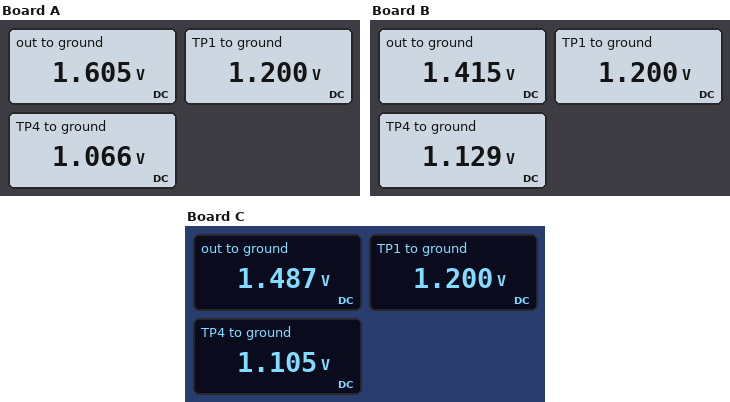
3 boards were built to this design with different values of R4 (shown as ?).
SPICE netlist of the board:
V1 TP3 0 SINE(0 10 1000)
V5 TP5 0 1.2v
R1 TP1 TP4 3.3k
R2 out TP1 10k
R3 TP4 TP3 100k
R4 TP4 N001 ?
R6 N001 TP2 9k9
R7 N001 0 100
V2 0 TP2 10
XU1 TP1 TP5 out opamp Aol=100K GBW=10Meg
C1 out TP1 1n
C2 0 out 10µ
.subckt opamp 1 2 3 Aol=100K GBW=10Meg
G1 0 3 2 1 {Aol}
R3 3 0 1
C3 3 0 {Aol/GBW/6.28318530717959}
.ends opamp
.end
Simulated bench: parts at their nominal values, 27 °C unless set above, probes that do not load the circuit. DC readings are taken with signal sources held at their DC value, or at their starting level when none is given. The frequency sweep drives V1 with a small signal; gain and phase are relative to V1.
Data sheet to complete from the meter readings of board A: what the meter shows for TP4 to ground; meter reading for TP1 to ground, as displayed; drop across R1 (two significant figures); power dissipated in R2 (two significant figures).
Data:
1.066 V
1.200 V
130 mV
16 µW
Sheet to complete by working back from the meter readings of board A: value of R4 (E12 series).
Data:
39 kΩ
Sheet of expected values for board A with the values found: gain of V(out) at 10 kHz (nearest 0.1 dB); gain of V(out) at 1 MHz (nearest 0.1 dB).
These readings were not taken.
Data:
-22.4 dB
-57.0 dB
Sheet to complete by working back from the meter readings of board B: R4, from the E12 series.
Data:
120 kΩ
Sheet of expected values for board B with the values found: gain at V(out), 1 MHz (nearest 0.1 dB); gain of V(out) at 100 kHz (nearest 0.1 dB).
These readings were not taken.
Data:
-56.5 dB
-36.6 dB
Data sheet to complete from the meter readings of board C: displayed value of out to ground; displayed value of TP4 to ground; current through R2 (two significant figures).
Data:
1.487 V
1.105 V
29 µA
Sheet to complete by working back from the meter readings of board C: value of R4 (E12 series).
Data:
68 kΩ
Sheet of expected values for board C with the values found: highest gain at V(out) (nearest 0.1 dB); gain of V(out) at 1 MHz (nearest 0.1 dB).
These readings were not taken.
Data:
-20.7 dB
-56.7 dB
